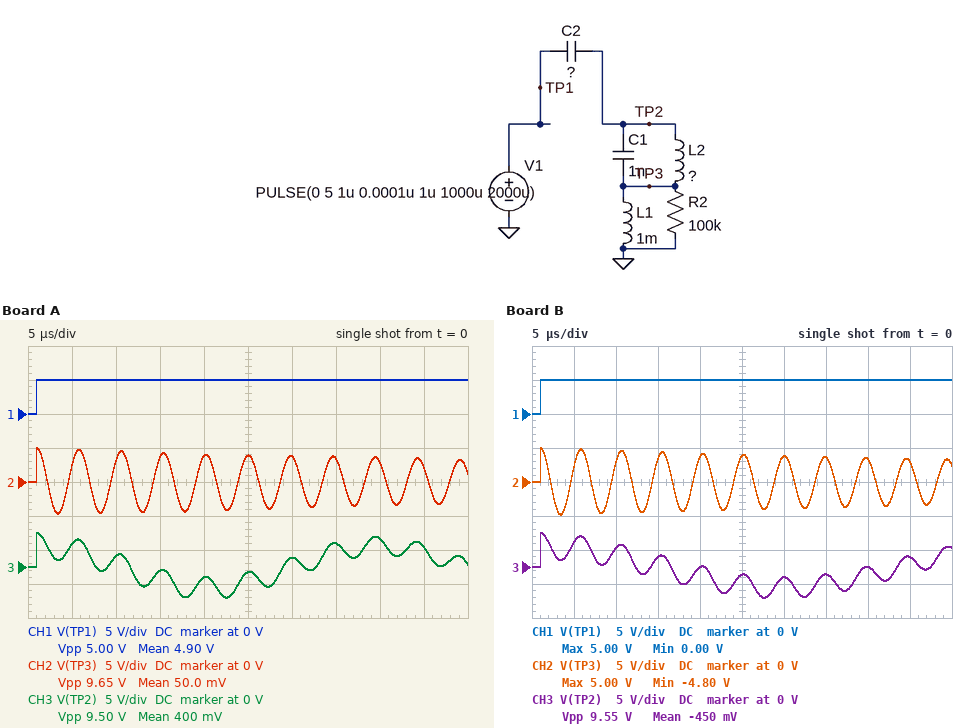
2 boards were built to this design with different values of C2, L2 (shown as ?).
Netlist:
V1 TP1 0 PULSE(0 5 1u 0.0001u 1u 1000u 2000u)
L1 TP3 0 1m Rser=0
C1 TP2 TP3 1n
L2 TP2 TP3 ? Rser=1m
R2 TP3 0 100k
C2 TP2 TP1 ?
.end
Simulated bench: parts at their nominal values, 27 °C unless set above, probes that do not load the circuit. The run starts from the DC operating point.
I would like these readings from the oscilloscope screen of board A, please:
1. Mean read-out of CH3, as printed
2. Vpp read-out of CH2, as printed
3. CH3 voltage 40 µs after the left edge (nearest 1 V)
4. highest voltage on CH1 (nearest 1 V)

400 mV
9.65 V
4 V
5 V
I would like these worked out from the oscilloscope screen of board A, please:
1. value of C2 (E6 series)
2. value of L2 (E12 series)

1.5 nF
15 mH
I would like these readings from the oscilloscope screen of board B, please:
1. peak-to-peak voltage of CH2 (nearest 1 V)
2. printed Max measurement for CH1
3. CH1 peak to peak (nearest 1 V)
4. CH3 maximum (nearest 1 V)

10 V
5.00 V
5 V
5 V
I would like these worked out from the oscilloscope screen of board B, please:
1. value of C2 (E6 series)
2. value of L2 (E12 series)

1.5 nF
33 mH
